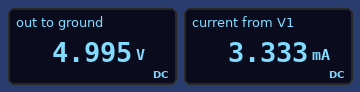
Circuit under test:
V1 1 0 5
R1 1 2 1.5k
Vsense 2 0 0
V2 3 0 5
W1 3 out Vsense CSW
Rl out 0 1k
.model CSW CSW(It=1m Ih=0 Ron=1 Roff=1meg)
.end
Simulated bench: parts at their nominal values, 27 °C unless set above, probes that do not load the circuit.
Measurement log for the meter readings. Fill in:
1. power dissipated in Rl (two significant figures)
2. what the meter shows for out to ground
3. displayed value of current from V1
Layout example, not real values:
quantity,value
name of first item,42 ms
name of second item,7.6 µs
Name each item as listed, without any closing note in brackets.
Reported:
quantity,value
power dissipated in Rl,25 mW
what the meter shows for out to ground,4.995 V
displayed value of current from V1,3.333 mA
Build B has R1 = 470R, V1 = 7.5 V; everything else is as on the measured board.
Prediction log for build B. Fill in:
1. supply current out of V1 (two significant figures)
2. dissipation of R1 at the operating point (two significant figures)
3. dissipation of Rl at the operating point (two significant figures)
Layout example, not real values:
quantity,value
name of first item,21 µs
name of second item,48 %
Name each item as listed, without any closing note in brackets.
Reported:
quantity,value
supply current out of V1,16 mA
dissipation of R1 at the operating point,120 mW
dissipation of Rl at the operating point,25 mW
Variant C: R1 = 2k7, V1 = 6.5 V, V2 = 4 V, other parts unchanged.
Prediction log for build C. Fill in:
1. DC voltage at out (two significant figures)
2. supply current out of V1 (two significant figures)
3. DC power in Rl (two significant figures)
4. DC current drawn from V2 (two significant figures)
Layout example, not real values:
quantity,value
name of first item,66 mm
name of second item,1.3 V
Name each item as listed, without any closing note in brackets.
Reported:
quantity,value
DC voltage at out,4.0 V
supply current out of V1,2.4 mA
DC power in Rl,16 mW
DC current drawn from V2,4.0 mA
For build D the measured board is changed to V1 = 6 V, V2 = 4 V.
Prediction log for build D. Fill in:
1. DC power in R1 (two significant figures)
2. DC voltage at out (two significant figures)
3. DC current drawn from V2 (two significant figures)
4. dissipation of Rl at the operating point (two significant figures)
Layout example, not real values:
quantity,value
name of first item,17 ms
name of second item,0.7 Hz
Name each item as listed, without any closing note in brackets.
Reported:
quantity,value
DC power in R1,24 mW
DC voltage at out,4.0 V
DC current drawn from V2,4.0 mA
dissipation of Rl at the operating point,16 mW
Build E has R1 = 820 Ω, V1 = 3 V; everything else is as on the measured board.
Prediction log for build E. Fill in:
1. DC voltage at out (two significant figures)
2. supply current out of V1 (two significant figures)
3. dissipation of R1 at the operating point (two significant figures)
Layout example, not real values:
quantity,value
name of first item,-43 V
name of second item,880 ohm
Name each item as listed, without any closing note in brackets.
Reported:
quantity,value
DC voltage at out,5.0 V
supply current out of V1,3.7 mA
dissipation of R1 at the operating point,11 mW
